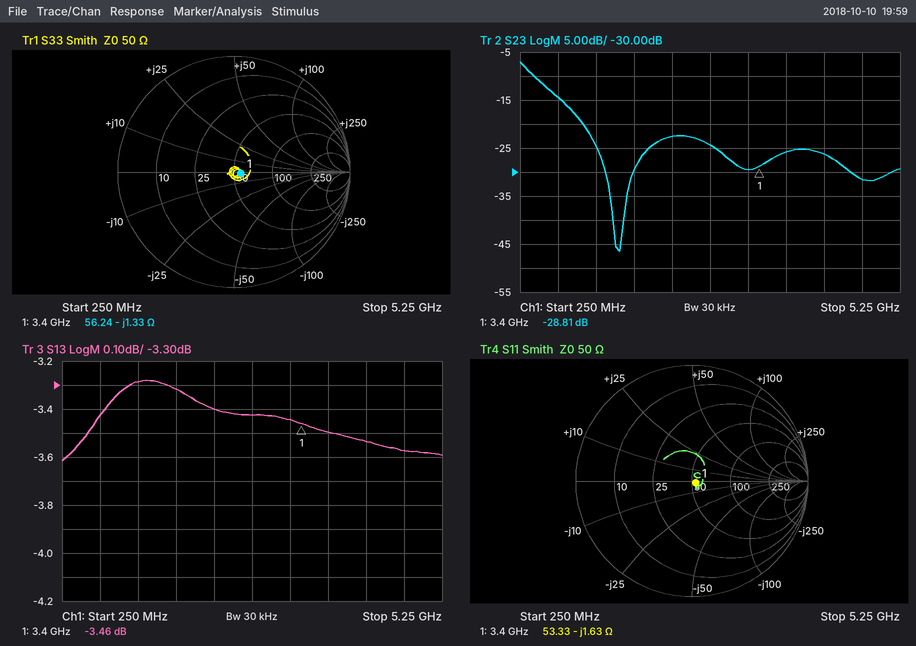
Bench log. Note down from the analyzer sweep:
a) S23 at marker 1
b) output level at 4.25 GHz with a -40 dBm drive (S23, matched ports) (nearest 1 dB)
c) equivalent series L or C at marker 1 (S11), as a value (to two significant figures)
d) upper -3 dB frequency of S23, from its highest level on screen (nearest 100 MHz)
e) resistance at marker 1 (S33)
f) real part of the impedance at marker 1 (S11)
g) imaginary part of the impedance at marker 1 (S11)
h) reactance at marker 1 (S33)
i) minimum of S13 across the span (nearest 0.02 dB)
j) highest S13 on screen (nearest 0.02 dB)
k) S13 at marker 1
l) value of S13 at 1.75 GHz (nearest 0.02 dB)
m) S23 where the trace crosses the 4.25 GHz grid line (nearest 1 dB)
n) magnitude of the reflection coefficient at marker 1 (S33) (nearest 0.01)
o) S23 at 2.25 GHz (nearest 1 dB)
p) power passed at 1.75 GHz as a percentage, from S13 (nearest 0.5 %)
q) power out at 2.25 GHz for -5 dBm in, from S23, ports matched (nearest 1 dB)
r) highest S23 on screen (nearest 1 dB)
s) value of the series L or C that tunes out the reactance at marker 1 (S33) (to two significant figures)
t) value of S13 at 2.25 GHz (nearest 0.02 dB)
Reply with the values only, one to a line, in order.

-28.81 dB
-66 dBm
29 pF
400 MHz
56.24 Ω
53.33 Ω
-1.63 Ω
-1.33 Ω
-3.62 dB
-3.28 dB
-3.46 dB
-3.32 dB
-26 dB
0.06
-23 dB
46.5 %
-28 dBm
-7 dB
62 pH
-3.40 dB
